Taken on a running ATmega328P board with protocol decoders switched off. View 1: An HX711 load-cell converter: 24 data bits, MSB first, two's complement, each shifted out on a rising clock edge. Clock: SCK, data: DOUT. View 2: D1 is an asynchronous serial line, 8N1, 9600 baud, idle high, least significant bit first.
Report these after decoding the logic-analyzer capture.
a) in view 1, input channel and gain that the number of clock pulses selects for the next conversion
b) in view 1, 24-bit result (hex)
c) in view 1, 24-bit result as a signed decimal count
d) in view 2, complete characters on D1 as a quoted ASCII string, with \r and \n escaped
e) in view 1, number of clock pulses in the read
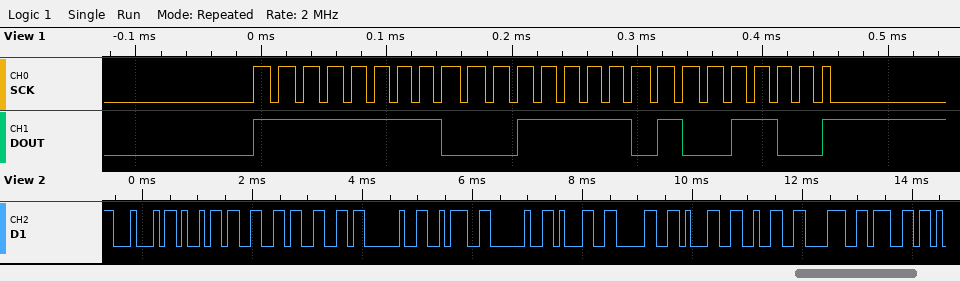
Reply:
channel A, gain 128
0xFF1F4C
-57524
"Diff : 10128g"
25
